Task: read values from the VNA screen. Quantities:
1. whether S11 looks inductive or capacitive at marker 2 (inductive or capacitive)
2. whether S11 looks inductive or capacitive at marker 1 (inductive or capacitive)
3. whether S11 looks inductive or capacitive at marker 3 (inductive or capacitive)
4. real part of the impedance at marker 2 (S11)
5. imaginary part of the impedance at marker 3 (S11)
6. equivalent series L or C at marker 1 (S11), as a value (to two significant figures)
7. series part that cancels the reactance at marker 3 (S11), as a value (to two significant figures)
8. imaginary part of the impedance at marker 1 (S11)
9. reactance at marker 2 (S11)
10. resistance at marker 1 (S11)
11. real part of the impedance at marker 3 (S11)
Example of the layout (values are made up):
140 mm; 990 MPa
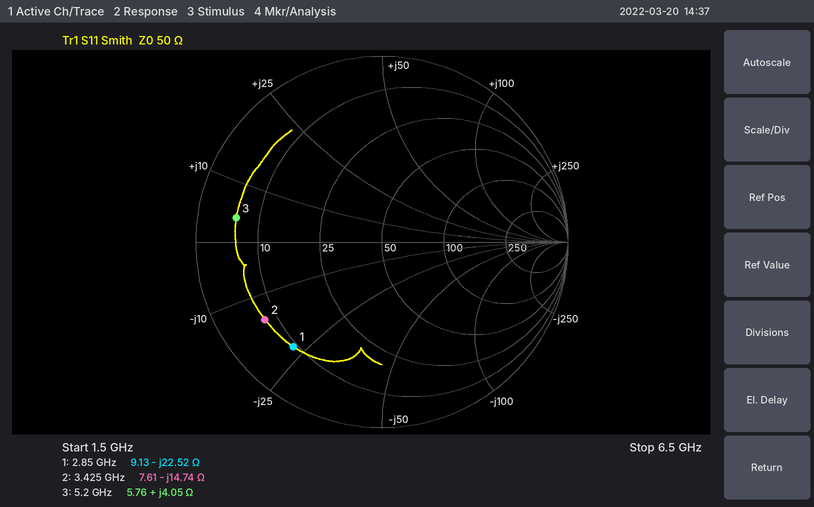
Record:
capacitive; capacitive; inductive; 7.61 Ω; +4.05 Ω; 2.5 pF; 7.6 pF; -22.52 Ω; -14.74 Ω; 9.13 Ω; 5.76 Ω
